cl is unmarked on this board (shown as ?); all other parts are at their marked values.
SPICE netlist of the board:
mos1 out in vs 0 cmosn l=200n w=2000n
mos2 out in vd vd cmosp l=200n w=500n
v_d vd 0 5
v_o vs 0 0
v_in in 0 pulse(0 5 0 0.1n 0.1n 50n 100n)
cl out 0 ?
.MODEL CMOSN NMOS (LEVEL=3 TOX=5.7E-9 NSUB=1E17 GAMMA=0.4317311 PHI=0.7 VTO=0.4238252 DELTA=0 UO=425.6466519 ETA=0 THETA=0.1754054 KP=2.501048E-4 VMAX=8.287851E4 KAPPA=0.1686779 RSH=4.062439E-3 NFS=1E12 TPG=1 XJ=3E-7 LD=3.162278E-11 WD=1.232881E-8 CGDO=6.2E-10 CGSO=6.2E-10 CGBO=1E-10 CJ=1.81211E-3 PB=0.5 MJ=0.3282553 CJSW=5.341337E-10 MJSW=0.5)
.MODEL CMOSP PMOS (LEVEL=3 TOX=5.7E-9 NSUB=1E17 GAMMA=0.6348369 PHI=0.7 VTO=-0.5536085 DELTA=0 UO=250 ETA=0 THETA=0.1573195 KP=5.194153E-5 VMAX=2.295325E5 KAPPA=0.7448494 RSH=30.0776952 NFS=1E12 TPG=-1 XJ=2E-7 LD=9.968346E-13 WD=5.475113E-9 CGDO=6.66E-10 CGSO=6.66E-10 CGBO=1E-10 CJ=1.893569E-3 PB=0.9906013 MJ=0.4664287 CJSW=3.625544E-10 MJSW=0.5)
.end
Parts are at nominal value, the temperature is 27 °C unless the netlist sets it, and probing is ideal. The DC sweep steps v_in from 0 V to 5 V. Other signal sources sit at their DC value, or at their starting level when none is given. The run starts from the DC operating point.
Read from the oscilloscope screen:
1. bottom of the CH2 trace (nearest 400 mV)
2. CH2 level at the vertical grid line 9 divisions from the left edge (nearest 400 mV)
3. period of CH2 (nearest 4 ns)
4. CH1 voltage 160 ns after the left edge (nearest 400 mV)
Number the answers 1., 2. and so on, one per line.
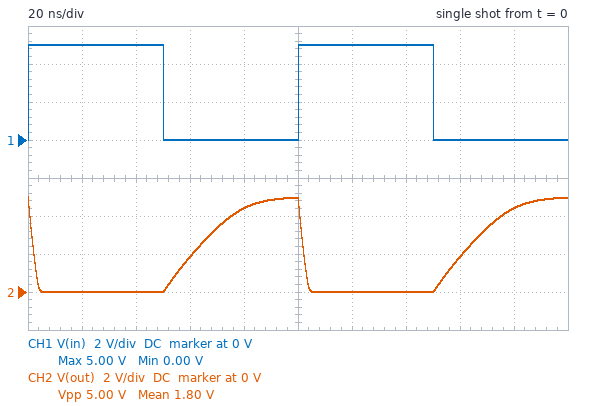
1. 0 V
2. 4.4 V
3. 100 ns
4. 0 V
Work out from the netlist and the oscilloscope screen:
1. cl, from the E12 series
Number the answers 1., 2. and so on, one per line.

1. 2.2 pF
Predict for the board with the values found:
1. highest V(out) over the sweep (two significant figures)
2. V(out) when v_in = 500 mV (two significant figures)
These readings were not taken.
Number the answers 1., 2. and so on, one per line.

1. 5.0 V
2. 4.7 V
